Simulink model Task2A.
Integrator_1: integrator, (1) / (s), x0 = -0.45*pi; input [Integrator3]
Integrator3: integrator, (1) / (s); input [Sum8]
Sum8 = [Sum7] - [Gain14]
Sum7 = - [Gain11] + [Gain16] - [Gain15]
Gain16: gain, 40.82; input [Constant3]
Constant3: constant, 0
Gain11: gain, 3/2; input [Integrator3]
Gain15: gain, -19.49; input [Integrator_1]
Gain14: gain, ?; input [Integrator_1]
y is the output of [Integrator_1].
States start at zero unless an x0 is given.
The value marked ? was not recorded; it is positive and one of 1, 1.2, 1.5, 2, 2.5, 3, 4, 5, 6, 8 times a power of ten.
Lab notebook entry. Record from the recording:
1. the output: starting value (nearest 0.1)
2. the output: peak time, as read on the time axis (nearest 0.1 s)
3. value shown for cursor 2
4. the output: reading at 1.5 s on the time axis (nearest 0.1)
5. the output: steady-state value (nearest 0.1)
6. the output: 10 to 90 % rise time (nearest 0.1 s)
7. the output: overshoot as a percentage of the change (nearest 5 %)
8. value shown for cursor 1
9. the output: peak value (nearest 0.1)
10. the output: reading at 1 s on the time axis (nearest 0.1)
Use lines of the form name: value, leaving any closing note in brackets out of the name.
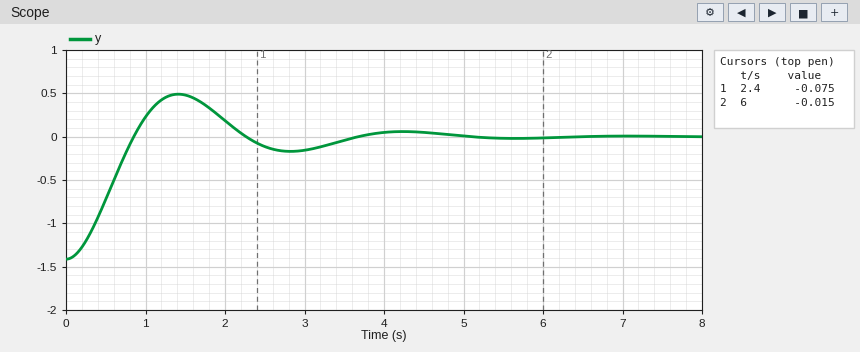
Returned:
the output: starting value: -1.4
the output: peak time, as read on the time axis: 1.4 s
value shown for cursor 2: -0.015
the output: reading at 1.5 s on the time axis: 0.5
the output: steady-state value: 0.0
the output: 10 to 90 % rise time: 0.6 s
the output: overshoot as a percentage of the change: 35 %
value shown for cursor 1: -0.075
the output: peak value: 0.5
the output: reading at 1 s on the time axis: 0.2
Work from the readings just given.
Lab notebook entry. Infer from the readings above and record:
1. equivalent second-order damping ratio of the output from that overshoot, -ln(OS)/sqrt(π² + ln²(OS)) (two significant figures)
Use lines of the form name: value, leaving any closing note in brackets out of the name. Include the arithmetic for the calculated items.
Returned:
equivalent second-order damping ratio of the output from that overshoot, -ln(OS)/sqrt(π² + ln²(OS)): ln(0.35) = -1.050; 1.050 / sqrt(9.870 + 1.102) = 0.32
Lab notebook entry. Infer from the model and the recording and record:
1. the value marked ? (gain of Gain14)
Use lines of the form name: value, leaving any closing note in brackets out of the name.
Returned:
the value marked ?: 25
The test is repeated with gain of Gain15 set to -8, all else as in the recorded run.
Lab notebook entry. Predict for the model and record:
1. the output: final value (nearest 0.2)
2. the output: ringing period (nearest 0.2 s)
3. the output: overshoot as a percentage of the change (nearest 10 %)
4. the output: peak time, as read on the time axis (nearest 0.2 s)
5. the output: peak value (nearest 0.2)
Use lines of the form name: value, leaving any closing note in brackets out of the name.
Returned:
the output: final value: 0.0
the output: ringing period: 1.6 s
the output: overshoot as a percentage of the change: 60 %
the output: peak time, as read on the time axis: 0.8 s
the output: peak value: 0.8
